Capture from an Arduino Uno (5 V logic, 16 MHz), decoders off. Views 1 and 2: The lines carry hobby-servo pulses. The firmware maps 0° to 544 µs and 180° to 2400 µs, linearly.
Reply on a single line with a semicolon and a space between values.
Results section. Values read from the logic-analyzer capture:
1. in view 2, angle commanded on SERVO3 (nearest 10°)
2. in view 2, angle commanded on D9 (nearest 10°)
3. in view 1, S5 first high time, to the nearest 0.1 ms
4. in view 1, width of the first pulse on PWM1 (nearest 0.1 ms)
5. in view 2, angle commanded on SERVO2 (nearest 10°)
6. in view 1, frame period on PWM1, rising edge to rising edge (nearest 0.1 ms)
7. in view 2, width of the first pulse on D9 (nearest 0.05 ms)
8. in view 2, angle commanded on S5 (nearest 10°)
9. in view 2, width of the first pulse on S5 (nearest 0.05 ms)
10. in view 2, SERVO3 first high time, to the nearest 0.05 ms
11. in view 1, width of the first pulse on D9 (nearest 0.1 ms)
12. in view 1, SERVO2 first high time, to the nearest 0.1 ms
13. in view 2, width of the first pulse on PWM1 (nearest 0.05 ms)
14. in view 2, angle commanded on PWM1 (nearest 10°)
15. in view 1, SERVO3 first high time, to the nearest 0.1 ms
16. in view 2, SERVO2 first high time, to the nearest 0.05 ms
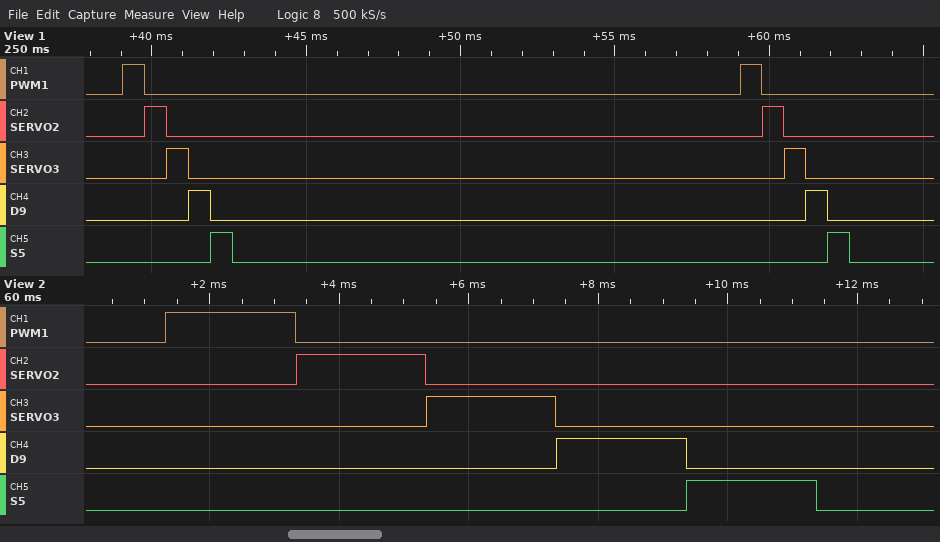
140°; 140°; 0.7 ms; 0.7 ms; 140°; 20.0 ms; 2.00 ms; 140°; 2.00 ms; 2.00 ms; 0.7 ms; 0.7 ms; 2.00 ms; 140°; 0.7 ms; 2.00 ms
